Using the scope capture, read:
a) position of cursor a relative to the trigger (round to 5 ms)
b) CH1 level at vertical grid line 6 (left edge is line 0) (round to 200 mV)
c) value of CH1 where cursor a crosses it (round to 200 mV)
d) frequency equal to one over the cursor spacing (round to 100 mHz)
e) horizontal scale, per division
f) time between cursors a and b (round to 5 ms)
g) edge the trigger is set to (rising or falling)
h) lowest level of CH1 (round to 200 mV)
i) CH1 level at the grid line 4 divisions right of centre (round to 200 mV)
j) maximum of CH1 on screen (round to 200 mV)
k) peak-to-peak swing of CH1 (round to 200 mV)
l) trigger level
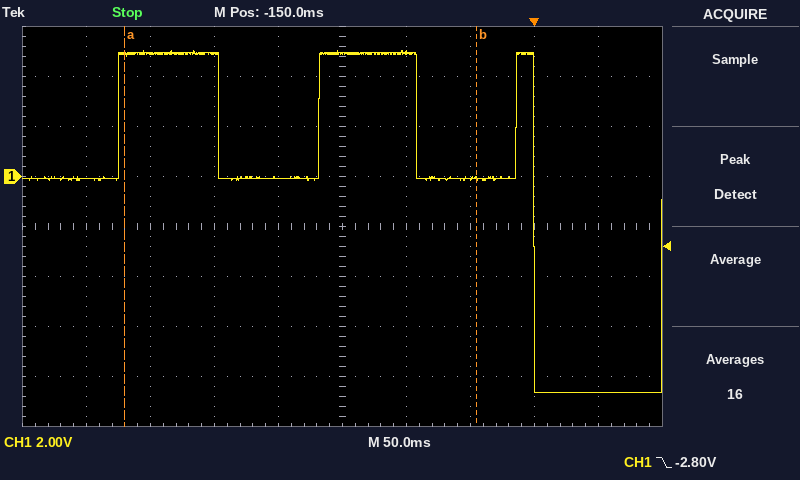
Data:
-320 ms
5.0 V
4.8 V
3.6 Hz
50 ms
275 ms
falling
-8.6 V
-8.6 V
5.0 V
13.6 V
-2.80 V
